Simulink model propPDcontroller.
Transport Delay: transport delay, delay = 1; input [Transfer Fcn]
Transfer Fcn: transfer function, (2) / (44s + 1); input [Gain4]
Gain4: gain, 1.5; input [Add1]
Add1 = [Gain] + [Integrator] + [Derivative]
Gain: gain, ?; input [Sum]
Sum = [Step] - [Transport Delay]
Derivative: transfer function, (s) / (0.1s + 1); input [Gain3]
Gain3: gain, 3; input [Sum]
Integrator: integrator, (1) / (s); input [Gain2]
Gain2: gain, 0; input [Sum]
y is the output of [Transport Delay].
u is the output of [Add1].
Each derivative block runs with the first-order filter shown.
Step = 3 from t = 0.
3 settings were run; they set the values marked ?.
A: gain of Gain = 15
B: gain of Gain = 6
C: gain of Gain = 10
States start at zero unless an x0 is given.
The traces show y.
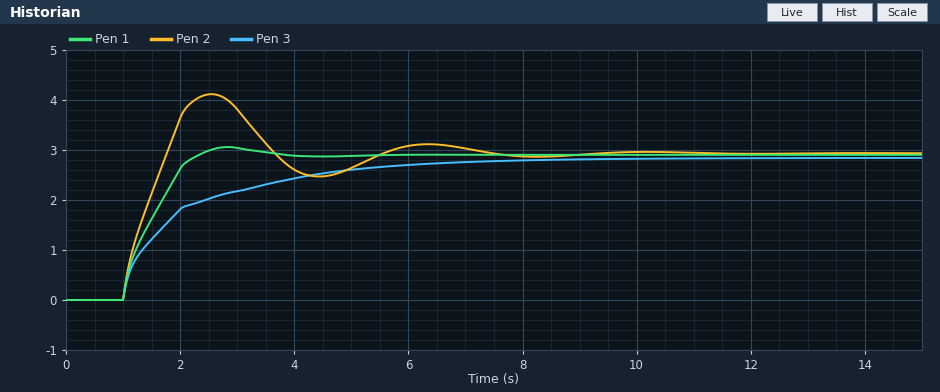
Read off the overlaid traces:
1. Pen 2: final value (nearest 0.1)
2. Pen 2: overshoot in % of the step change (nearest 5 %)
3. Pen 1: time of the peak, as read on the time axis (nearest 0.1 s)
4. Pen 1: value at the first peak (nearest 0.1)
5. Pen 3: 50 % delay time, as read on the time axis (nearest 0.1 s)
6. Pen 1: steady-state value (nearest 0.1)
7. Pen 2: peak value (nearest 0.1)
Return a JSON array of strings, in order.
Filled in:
["2.9", "40 %", "2.8 s", "3.1", "1.7 s", "2.9", "4.1"]
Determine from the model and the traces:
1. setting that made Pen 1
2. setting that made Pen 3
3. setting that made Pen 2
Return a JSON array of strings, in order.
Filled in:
["C", "B", "A"]
